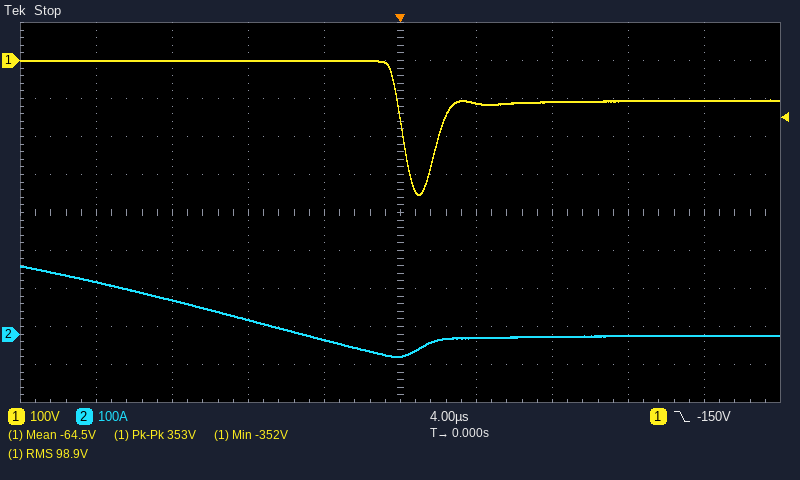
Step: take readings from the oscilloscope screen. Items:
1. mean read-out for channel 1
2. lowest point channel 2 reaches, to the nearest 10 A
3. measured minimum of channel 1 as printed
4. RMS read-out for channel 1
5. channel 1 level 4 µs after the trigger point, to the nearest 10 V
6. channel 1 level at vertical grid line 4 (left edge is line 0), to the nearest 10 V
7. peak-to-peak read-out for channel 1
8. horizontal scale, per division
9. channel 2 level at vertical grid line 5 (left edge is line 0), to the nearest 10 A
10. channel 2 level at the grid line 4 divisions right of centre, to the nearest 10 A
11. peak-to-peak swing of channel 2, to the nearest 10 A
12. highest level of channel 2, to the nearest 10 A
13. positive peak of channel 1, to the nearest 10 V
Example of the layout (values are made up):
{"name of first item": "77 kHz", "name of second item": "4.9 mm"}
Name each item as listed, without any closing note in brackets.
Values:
{"mean read-out for channel 1": "-64.5 V", "lowest point channel 2 reaches, to the nearest 10 A": "-60 A", "measured minimum of channel 1 as printed": "-352 V", "RMS read-out for channel 1": "98.9 V", "channel 1 level 4 µs after the trigger point, to the nearest 10 V": "-110 V", "channel 1 level at vertical grid line 4 (left edge is line 0), to the nearest 10 V": "0 V", "peak-to-peak read-out for channel 1": "353 V", "horizontal scale, per division": "4 µs", "channel 2 level at vertical grid line 5 (left edge is line 0), to the nearest 10 A": "-60 A", "channel 2 level at the grid line 4 divisions right of centre, to the nearest 10 A": "0 A", "peak-to-peak swing of channel 2, to the nearest 10 A": "240 A", "highest level of channel 2, to the nearest 10 A": "180 A", "positive peak of channel 1, to the nearest 10 V": "0 V"}
